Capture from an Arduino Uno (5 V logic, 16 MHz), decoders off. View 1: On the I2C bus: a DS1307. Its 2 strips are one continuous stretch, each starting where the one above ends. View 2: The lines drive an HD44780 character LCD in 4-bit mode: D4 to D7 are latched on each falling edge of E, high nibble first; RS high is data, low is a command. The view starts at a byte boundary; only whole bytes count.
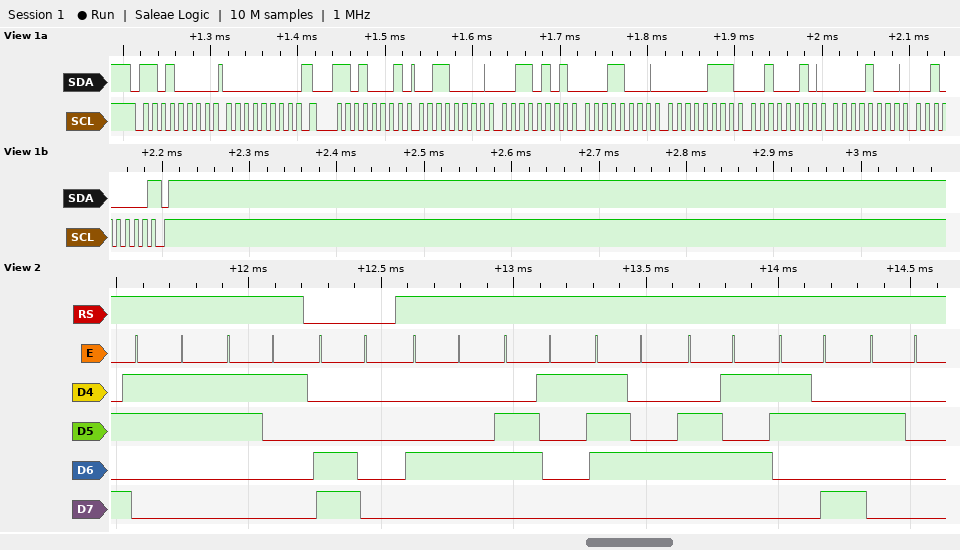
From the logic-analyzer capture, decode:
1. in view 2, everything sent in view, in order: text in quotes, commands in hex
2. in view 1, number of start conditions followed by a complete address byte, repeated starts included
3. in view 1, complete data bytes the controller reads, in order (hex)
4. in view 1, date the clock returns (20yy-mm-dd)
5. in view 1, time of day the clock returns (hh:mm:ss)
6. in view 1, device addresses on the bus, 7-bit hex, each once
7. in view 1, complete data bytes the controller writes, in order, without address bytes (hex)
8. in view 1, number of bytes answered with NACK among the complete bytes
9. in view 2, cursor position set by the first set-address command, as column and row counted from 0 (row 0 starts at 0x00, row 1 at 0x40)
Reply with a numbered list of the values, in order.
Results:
1. "31" 0xC0 "Date: "
2. 2
3. 30 35 18 07 22 08 20
4. 2020-08-22
5. 18:35:30
6. 0x68
7. 00
8. 1
9. column 0, row 1
